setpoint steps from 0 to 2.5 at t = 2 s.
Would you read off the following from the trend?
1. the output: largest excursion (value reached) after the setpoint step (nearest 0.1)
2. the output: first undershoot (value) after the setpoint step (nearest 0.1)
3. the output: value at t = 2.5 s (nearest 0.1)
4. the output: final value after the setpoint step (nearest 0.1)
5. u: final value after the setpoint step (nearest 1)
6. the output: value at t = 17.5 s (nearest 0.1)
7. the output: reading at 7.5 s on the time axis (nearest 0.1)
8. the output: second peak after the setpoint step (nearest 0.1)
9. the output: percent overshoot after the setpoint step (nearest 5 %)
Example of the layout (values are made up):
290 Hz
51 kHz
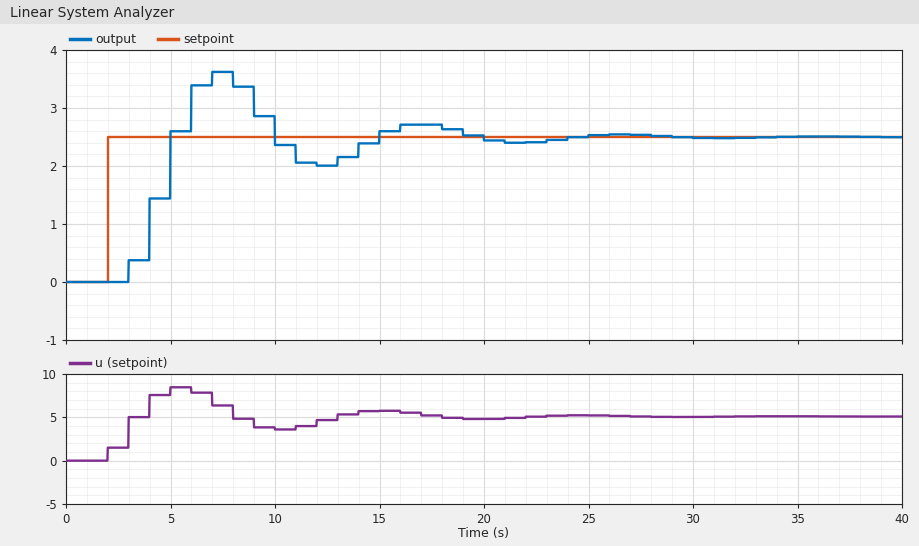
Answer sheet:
3.6
2.0
0.0
2.5
5
2.7
3.6
2.7
45 %
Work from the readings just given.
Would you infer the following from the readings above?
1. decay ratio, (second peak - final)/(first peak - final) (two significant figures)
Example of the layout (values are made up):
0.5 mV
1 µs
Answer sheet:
0.18
